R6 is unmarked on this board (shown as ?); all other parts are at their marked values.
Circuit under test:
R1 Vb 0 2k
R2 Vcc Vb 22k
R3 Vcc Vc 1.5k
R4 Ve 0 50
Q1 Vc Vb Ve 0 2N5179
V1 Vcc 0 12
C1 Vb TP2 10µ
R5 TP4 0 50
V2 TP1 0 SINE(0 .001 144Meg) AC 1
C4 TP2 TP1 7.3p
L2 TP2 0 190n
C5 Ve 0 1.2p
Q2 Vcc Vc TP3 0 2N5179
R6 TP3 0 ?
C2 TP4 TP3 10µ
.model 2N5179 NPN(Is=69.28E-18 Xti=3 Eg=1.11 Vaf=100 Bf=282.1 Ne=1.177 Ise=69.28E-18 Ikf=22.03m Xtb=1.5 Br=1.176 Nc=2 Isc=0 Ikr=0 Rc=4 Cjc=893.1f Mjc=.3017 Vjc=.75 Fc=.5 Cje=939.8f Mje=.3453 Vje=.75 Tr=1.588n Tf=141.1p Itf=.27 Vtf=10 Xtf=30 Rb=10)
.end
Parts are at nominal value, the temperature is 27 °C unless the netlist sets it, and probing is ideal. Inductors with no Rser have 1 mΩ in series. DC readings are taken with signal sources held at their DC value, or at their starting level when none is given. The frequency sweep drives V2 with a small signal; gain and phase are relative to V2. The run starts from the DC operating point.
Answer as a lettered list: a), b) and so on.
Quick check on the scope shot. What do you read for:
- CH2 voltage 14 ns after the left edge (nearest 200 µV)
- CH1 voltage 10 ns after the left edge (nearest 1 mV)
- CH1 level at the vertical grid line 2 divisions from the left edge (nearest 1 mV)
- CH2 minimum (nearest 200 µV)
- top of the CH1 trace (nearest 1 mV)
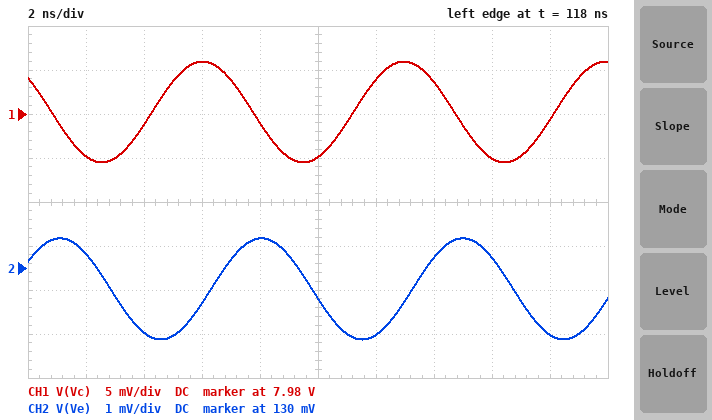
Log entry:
a) 130.2 mV
b) 7.975 V
c) 7.979 V
d) 128.4 mV
e) 7.986 V
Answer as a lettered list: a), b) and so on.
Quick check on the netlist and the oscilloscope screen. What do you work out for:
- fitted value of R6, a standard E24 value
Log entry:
a) 820 Ω
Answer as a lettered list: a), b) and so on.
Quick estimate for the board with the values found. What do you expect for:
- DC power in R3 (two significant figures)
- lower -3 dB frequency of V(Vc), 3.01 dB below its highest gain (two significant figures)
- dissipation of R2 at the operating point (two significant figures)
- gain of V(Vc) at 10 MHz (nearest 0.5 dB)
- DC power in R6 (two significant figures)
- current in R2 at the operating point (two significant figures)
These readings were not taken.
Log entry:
a) 11 mW
b) 93 MHz
c) 5.6 mW
d) -21.0 dB
e) 62 mW
f) 500 µA
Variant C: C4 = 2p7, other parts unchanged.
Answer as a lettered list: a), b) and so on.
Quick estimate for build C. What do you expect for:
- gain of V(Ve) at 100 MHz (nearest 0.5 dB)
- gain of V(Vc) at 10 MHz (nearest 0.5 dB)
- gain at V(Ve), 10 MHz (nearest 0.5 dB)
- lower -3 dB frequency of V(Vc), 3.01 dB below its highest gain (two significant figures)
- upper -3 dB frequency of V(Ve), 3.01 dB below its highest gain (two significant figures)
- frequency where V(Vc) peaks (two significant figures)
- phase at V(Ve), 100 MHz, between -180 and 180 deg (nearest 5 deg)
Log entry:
a) -11.0 dB
b) -30.0 dB
c) -55.5 dB
d) 120 MHz
e) 230 MHz
f) 150 MHz
g) 150 deg
